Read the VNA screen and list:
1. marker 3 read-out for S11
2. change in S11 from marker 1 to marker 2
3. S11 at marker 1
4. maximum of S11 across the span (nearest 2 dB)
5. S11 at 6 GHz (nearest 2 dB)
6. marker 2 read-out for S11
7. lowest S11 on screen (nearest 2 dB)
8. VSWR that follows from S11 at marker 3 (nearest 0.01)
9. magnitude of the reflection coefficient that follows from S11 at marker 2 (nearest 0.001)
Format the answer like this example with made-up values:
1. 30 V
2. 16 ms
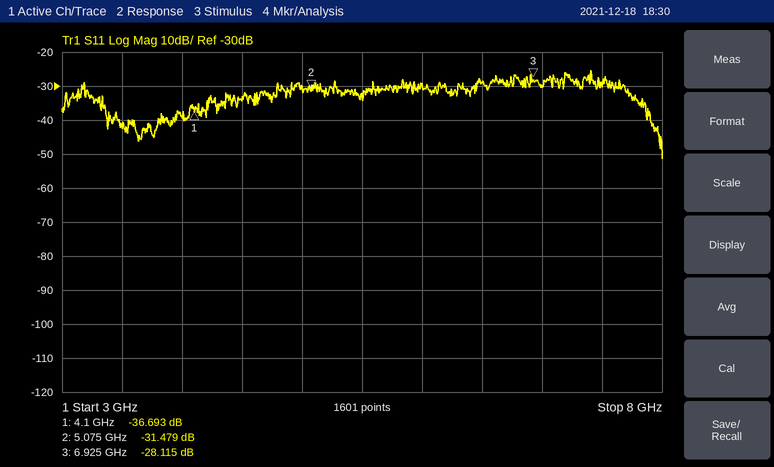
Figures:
1. -28.115 dB
2. 5.214 dB
3. -36.693 dB
4. -26 dB
5. -30 dB
6. -31.479 dB
7. -52 dB
8. 1.08
9. 0.027
